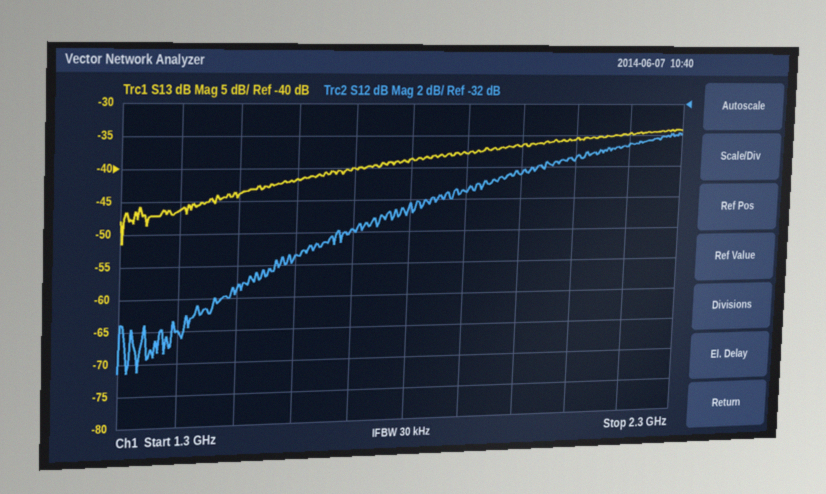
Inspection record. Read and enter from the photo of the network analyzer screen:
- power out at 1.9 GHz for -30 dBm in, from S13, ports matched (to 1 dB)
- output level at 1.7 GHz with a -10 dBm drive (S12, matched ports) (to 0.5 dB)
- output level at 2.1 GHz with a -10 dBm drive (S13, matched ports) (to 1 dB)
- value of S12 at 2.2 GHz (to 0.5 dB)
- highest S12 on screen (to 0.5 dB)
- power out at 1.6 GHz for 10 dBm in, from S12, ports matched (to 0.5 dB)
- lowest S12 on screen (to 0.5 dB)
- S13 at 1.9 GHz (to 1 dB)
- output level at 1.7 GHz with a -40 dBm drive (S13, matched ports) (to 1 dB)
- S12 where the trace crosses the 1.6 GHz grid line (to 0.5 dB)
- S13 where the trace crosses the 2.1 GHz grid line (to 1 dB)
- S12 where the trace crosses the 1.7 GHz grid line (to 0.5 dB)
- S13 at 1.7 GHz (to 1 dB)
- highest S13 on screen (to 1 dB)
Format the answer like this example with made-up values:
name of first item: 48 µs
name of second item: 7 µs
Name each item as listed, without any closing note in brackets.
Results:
power out at 1.9 GHz for -30 dBm in, from S13, ports matched: -68 dBm
output level at 1.7 GHz with a -10 dBm drive (S12, matched ports): -50.0 dBm
output level at 2.1 GHz with a -10 dBm drive (S13, matched ports): -46 dBm
value of S12 at 2.2 GHz: -34.5 dB
highest S12 on screen: -34.0 dB
power out at 1.6 GHz for 10 dBm in, from S12, ports matched: -31.5 dBm
lowest S12 on screen: -48.5 dB
S13 at 1.9 GHz: -38 dB
output level at 1.7 GHz with a -40 dBm drive (S13, matched ports): -80 dBm
S12 where the trace crosses the 1.6 GHz grid line: -41.5 dB
S13 where the trace crosses the 2.1 GHz grid line: -36 dB
S12 where the trace crosses the 1.7 GHz grid line: -40.0 dB
S13 at 1.7 GHz: -40 dB
highest S13 on screen: -34 dB
